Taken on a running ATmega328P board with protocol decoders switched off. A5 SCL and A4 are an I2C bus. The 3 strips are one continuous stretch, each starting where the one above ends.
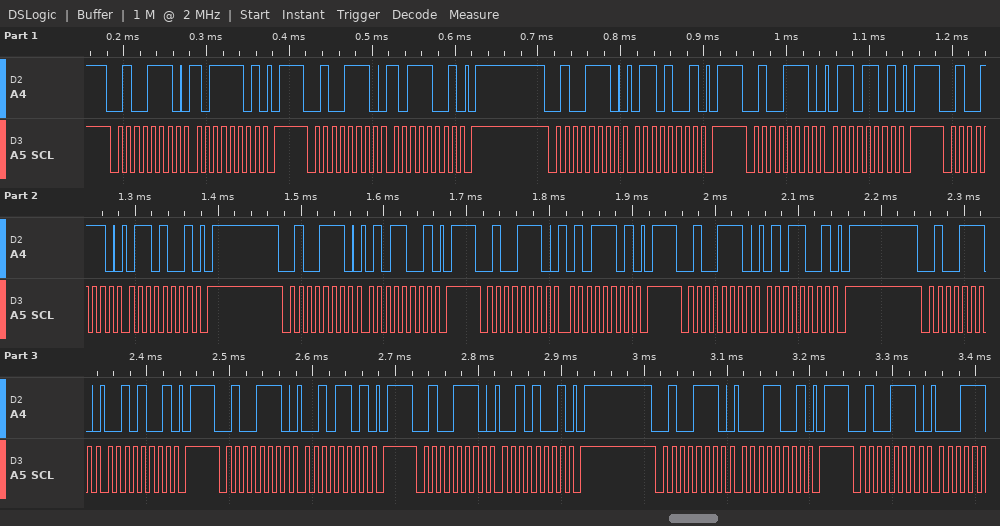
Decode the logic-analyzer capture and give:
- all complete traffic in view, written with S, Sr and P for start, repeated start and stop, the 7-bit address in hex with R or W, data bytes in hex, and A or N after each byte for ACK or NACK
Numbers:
S 27W A BD A P S 27W A B9 A P S 27W A 69 A P S 27W A 6D A P S 27W A 69 A P S 27W A 59 A P S 27W A 5D A P S 27W A 59 A P S 27W A 29 A P S 27W A 2D A P S 27W A 29 A P S 27W A 19 A P S 27W A
